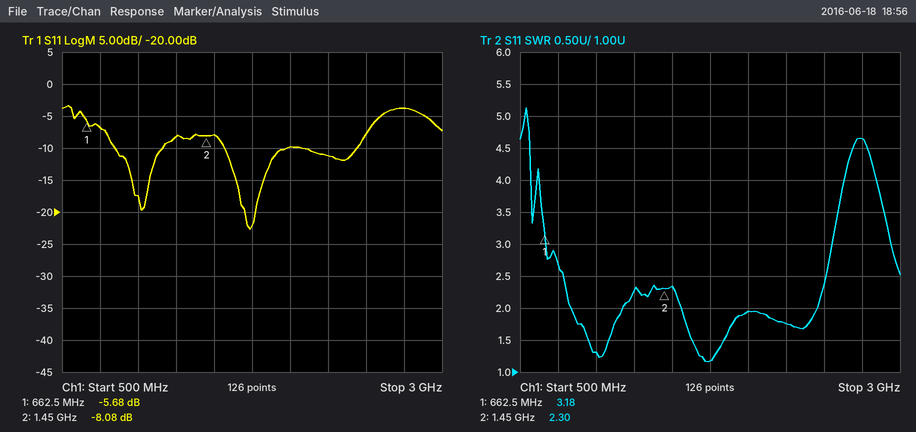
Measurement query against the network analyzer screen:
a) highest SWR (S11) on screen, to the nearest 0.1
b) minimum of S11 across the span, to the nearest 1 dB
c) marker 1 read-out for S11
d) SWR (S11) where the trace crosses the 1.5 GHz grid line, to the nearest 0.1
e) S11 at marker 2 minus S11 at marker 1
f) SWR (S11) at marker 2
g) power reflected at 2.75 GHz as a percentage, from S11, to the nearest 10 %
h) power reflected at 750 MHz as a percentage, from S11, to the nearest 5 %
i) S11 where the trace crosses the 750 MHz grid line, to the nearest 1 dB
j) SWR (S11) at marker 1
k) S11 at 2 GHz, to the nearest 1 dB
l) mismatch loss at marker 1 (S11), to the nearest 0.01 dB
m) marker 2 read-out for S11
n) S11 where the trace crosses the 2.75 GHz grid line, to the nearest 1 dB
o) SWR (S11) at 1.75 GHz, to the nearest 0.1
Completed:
5.1
-23 dB
-5.68 dB
2.3
-2.40 dB
2.30
40 %
20 %
-7 dB
3.18
-10 dB
1.37 dB
-8.08 dB
-4 dB
1.2
